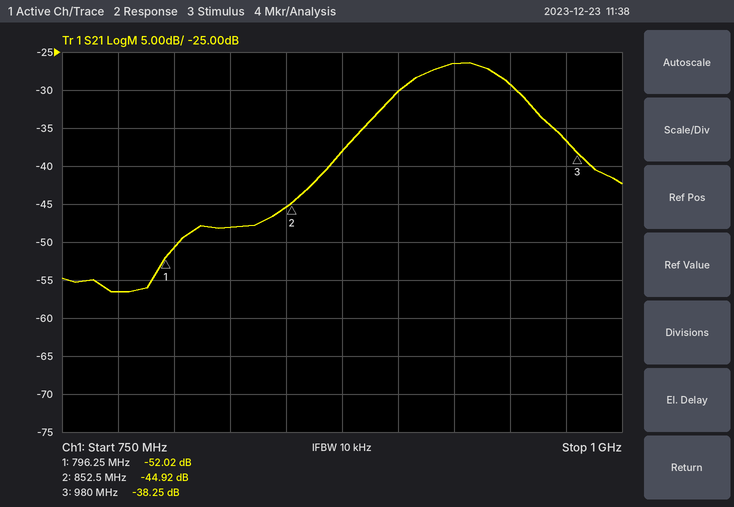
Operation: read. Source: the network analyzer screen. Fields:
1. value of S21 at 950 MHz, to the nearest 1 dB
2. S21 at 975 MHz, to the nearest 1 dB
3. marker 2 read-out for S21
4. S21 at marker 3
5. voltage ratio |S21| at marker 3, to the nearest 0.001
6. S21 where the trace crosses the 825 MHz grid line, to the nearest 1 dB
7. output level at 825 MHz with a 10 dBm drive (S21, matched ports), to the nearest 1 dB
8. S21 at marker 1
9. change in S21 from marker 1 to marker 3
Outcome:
-29 dB
-37 dB
-44.92 dB
-38.25 dB
0.012
-48 dB
-38 dBm
-52.02 dB
13.77 dB
